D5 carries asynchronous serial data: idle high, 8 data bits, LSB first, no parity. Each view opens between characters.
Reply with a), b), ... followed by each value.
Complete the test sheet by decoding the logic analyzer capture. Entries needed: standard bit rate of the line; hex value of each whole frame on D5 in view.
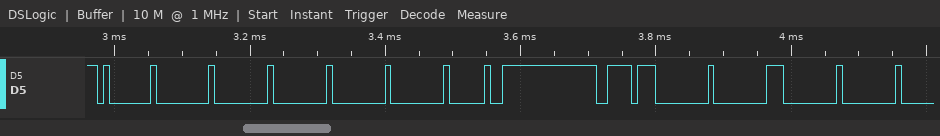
a) 115200 baud
b) 01, 00, 00, 00, 00, 00, 20, DE, 00, 00, 00, 00
